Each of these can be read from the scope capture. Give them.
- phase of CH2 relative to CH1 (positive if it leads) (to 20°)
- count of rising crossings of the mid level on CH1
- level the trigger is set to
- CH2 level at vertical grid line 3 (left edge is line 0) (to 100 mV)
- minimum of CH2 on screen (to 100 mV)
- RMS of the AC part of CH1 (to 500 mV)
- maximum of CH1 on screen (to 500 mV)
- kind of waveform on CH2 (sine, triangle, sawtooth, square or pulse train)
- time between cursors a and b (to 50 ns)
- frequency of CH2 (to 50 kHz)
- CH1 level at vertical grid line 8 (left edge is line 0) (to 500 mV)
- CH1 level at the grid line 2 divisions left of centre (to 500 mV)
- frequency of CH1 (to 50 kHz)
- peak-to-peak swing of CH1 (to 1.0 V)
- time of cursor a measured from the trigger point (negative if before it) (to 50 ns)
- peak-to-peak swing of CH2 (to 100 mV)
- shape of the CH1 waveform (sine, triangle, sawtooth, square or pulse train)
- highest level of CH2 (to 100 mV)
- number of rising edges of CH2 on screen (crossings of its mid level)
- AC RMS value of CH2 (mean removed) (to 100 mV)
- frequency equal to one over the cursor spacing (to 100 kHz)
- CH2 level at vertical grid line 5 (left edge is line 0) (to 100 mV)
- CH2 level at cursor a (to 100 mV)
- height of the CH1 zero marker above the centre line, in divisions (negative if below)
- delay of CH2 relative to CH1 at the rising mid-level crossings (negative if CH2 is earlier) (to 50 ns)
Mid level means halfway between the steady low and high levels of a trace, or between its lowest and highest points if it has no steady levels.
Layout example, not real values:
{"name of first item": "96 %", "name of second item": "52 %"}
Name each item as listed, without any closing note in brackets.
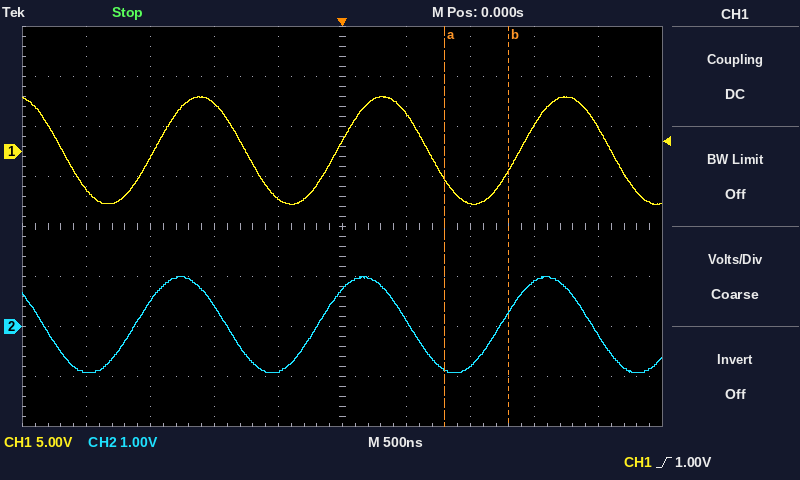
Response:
{"phase of CH2 relative to CH1 (positive if it leads)": "+40°", "count of rising crossings of the mid level on CH1": "3", "level the trigger is set to": "1.00 V", "CH2 level at vertical grid line 3 (left edge is line 0)": "400 mV", "minimum of CH2 on screen": "-900 mV", "RMS of the AC part of CH1": "4.0 V", "maximum of CH1 on screen": "5.5 V", "kind of waveform on CH2": "sine", "time between cursors a and b": "500 ns", "frequency of CH2": "700 kHz", "CH1 level at vertical grid line 8 (left edge is line 0)": "2.5 V", "CH1 level at the grid line 2 divisions left of centre": "5.0 V", "frequency of CH1": "700 kHz", "peak-to-peak swing of CH1": "11.0 V", "time of cursor a measured from the trigger point (negative if before it)": "+800 ns", "peak-to-peak swing of CH2": "1.9 V", "shape of the CH1 waveform": "sine", "highest level of CH2": "1.0 V", "number of rising edges of CH2 on screen": "3", "AC RMS value of CH2 (mean removed)": "700 mV", "frequency equal to one over the cursor spacing": "2.0 MHz", "CH2 level at vertical grid line 5 (left edge is line 0)": "700 mV", "CH2 level at cursor a": "-900 mV", "height of the CH1 zero marker above the centre line, in divisions": "+1.5 div", "delay of CH2 relative to CH1 at the rising mid-level crossings (negative if CH2 is earlier)": "-150 ns"}
